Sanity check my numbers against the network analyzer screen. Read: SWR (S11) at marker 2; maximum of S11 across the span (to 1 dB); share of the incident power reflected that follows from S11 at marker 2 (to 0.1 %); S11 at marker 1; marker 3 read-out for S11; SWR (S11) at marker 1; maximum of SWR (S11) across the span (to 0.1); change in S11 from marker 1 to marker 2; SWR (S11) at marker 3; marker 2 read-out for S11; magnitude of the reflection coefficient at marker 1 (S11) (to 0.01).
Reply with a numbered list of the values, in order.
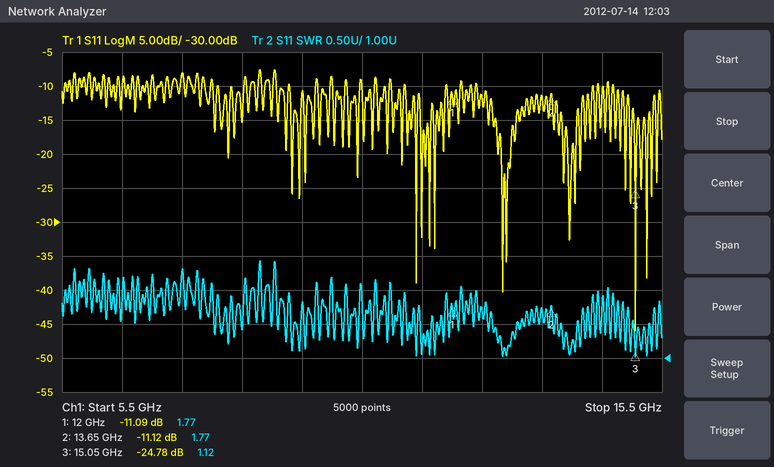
1. 1.77
2. -8 dB
3. 7.7 %
4. -11.09 dB
5. -24.78 dB
6. 1.77
7. 2.4
8. -0.03 dB
9. 1.12
10. -11.12 dB
11. 0.28
